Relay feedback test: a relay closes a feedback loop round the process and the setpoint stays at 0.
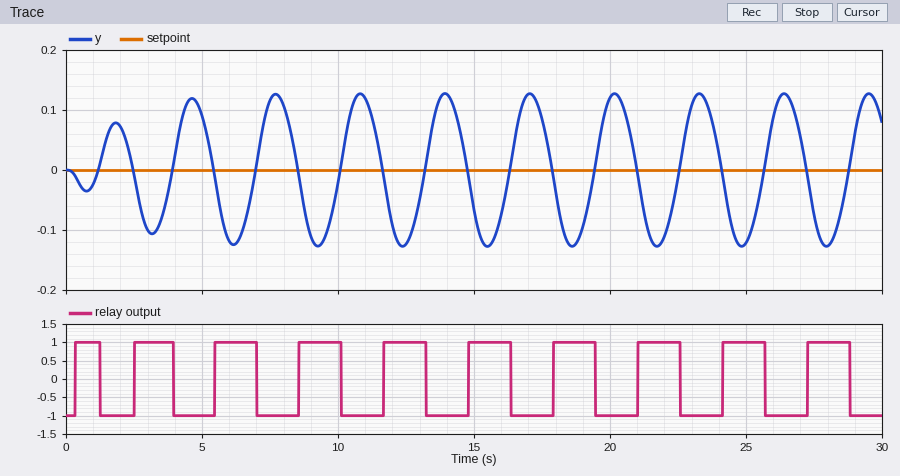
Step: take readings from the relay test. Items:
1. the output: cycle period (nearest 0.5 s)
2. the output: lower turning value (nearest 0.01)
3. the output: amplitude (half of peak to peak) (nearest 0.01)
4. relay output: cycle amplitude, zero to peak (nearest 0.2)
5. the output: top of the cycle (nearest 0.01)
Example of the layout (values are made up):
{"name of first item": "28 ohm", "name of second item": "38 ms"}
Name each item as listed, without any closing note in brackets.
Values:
{"the output: cycle period": "3.0 s", "the output: lower turning value": "-0.13", "the output: amplitude (half of peak to peak)": "0.13", "relay output: cycle amplitude, zero to peak": "1.0", "the output: top of the cycle": "0.13"}
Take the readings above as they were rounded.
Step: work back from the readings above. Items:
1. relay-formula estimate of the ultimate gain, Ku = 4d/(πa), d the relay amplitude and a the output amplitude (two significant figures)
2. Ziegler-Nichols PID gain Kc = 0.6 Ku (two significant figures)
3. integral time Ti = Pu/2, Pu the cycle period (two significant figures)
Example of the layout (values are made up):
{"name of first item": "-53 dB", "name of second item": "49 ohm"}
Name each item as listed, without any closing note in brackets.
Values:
{"relay-formula estimate of the ultimate gain, Ku = 4d/(πa), d the relay amplitude and a the output amplitude": "9.8", "Ziegler-Nichols PID gain Kc = 0.6 Ku": "5.9", "integral time Ti = Pu/2, Pu the cycle period": "1.5 s"}
